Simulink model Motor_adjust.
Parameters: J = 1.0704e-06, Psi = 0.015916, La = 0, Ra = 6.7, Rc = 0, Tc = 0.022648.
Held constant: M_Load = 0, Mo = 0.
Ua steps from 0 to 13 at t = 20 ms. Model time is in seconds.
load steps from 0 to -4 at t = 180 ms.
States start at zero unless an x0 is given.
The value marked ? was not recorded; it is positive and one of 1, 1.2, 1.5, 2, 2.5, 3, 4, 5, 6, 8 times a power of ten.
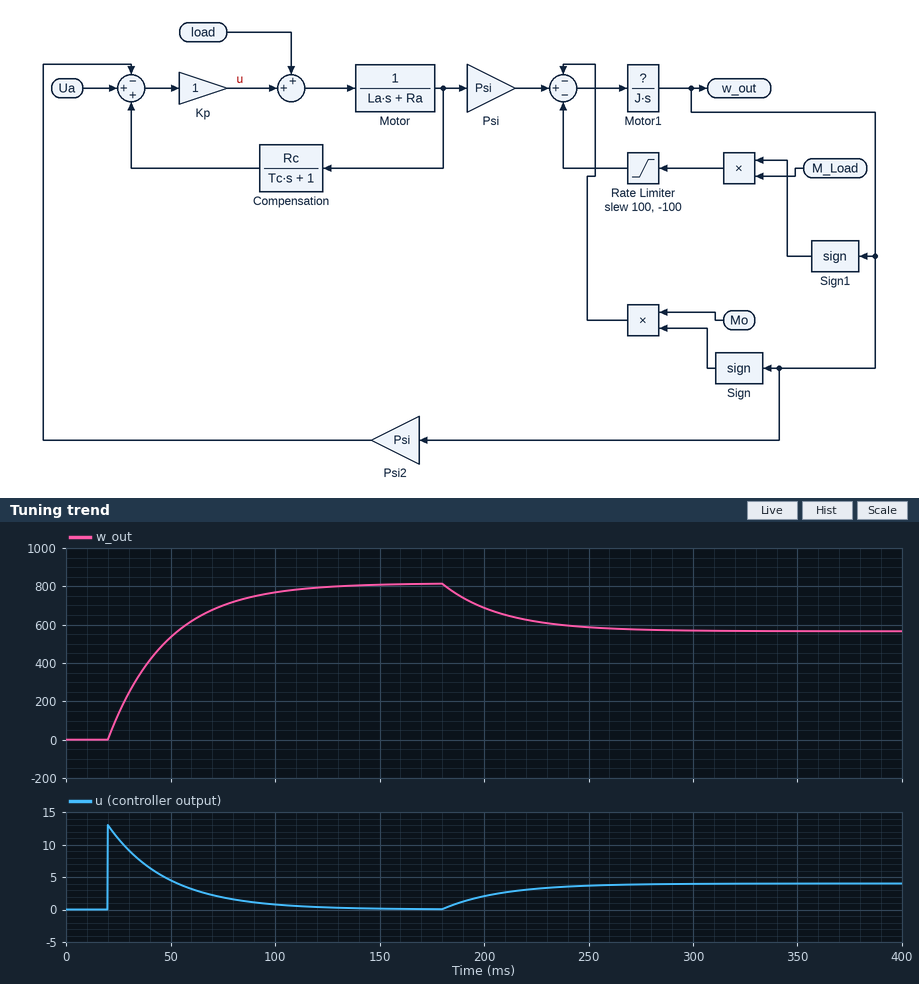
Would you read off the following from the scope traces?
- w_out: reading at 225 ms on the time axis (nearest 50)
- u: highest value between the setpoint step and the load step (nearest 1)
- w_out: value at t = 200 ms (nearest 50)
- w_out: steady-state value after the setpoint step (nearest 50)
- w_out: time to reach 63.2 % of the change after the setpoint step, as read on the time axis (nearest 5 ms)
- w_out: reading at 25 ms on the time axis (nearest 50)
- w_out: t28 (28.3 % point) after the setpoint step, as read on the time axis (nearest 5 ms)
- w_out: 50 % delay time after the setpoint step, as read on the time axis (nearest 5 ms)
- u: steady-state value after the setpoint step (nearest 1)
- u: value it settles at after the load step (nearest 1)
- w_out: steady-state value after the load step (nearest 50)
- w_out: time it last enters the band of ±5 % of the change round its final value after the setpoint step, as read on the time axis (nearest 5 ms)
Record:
600
13
700
800
50 ms
150
30 ms
40 ms
0
4
550
105 ms
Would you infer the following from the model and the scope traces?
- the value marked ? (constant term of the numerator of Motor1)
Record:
1
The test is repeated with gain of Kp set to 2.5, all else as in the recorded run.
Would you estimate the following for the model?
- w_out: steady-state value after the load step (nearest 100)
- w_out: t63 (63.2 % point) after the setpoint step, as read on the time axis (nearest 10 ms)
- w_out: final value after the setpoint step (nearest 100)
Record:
700
30 ms
800
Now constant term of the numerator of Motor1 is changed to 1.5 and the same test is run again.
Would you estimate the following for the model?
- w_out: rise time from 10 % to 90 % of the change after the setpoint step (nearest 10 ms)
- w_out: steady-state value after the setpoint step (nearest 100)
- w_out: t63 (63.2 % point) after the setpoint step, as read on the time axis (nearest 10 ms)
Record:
40 ms
800
40 ms
